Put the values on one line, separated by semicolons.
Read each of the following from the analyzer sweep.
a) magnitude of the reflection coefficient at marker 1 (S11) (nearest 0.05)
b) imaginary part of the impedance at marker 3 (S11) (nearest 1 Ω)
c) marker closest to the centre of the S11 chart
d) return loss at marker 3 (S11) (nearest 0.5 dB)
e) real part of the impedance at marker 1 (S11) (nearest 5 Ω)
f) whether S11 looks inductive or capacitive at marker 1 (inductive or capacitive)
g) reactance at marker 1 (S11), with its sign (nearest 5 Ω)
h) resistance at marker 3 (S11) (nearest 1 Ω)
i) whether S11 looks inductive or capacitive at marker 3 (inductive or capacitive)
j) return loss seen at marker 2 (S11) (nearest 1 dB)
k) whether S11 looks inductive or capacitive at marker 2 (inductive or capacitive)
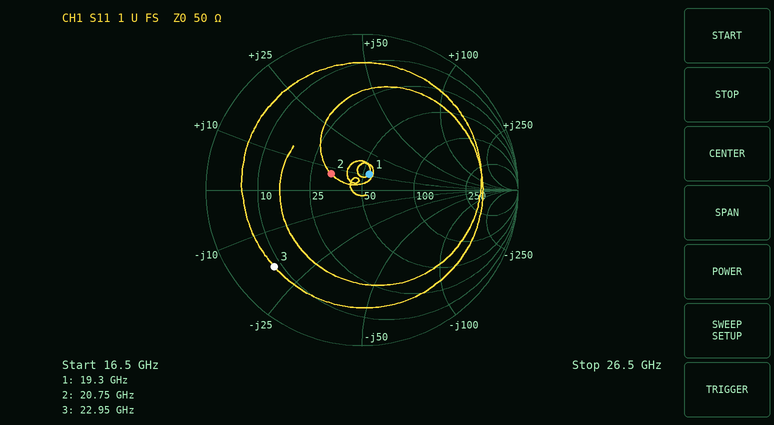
0.10; -18 Ω; marker 1; 2.5 dB; 55 Ω; inductive; +10 Ω; 8 Ω; capacitive; 13 dB; inductive
